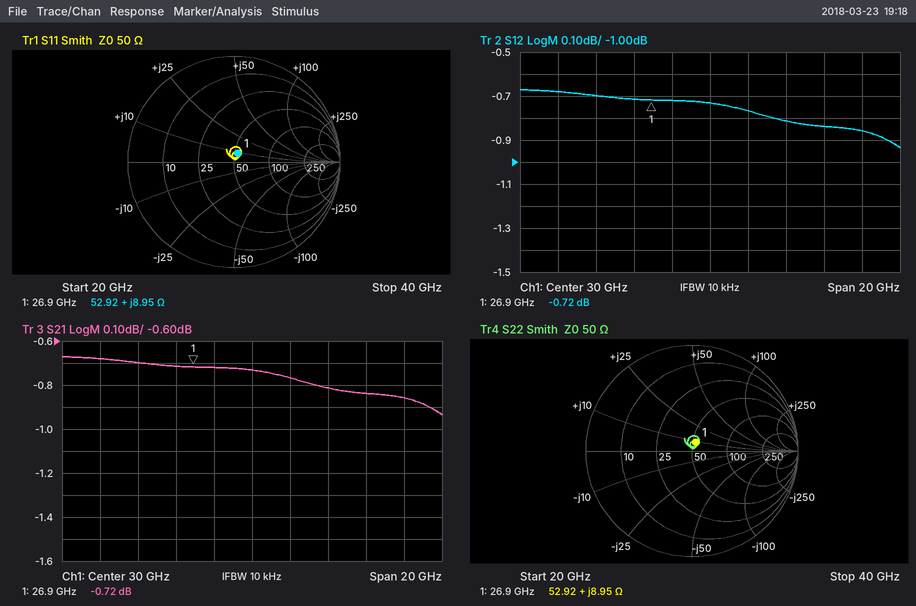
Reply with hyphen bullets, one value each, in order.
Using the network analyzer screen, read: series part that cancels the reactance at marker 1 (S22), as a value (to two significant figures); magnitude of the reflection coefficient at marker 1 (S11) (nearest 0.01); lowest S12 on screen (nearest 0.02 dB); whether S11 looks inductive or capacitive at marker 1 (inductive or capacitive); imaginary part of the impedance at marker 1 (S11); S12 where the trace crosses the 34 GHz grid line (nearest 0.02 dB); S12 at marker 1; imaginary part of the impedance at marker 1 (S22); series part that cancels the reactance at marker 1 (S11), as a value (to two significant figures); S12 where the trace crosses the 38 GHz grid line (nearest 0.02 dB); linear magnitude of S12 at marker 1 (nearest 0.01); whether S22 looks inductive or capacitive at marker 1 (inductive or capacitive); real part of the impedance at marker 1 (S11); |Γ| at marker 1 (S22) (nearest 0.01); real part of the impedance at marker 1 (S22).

- 660 fF
- 0.09
- -0.94 dB
- inductive
- +8.95 Ω
- -0.82 dB
- -0.72 dB
- +8.95 Ω
- 660 fF
- -0.86 dB
- 0.92
- inductive
- 52.92 Ω
- 0.09
- 52.92 Ω
